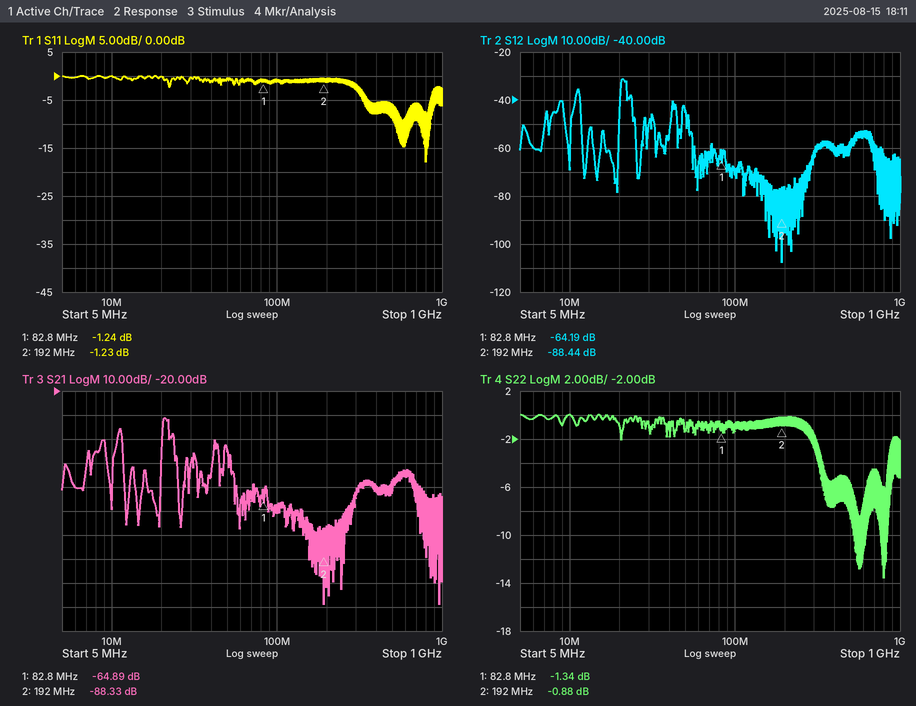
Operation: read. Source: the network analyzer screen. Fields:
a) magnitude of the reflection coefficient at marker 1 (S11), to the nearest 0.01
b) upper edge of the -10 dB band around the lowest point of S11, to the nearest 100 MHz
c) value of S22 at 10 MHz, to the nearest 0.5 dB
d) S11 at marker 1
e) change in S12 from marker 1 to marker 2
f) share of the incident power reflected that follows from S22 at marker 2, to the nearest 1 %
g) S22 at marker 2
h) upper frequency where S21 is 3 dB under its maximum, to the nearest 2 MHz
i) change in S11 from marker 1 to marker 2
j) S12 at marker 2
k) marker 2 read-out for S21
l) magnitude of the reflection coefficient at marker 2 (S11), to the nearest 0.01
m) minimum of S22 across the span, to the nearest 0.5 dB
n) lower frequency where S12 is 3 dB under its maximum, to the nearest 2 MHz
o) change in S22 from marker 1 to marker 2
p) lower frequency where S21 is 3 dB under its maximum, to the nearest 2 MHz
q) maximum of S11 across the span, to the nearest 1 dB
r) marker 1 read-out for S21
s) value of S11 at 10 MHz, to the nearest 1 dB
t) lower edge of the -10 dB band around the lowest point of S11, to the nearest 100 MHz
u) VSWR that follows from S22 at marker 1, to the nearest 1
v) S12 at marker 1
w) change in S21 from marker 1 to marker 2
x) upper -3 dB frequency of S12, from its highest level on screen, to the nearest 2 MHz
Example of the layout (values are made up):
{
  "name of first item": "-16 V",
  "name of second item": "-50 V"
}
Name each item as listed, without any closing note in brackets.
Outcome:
{
  "magnitude of the reflection coefficient at marker 1 (S11), to the nearest 0.01": "0.87",
  "upper edge of the -10 dB band around the lowest point of S11, to the nearest 100 MHz": "800 MHz",
  "value of S22 at 10 MHz, to the nearest 0.5 dB": "0.0 dB",
  "S11 at marker 1": "-1.24 dB",
  "change in S12 from marker 1 to marker 2": "-24.25 dB",
  "share of the incident power reflected that follows from S22 at marker 2, to the nearest 1 %": "82 %",
  "S22 at marker 2": "-0.88 dB",
  "upper frequency where S21 is 3 dB under its maximum, to the nearest 2 MHz": "22 MHz",
  "change in S11 from marker 1 to marker 2": "0.01 dB",
  "S12 at marker 2": "-88.44 dB",
  "marker 2 read-out for S21": "-88.33 dB",
  "magnitude of the reflection coefficient at marker 2 (S11), to the nearest 0.01": "0.87",
  "minimum of S22 across the span, to the nearest 0.5 dB": "-13.5 dB",
  "lower frequency where S12 is 3 dB under its maximum, to the nearest 2 MHz": "20 MHz",
  "change in S22 from marker 1 to marker 2": "0.46 dB",
  "lower frequency where S21 is 3 dB under its maximum, to the nearest 2 MHz": "20 MHz",
  "maximum of S11 across the span, to the nearest 1 dB": "0 dB",
  "marker 1 read-out for S21": "-64.89 dB",
  "value of S11 at 10 MHz, to the nearest 1 dB": "0 dB",
  "lower edge of the -10 dB band around the lowest point of S11, to the nearest 100 MHz": "800 MHz",
  "VSWR that follows from S22 at marker 1, to the nearest 1": "13",
  "S12 at marker 1": "-64.19 dB",
  "change in S21 from marker 1 to marker 2": "-23.44 dB",
  "upper -3 dB frequency of S12, from its highest level on screen, to the nearest 2 MHz": "22 MHz"
}
